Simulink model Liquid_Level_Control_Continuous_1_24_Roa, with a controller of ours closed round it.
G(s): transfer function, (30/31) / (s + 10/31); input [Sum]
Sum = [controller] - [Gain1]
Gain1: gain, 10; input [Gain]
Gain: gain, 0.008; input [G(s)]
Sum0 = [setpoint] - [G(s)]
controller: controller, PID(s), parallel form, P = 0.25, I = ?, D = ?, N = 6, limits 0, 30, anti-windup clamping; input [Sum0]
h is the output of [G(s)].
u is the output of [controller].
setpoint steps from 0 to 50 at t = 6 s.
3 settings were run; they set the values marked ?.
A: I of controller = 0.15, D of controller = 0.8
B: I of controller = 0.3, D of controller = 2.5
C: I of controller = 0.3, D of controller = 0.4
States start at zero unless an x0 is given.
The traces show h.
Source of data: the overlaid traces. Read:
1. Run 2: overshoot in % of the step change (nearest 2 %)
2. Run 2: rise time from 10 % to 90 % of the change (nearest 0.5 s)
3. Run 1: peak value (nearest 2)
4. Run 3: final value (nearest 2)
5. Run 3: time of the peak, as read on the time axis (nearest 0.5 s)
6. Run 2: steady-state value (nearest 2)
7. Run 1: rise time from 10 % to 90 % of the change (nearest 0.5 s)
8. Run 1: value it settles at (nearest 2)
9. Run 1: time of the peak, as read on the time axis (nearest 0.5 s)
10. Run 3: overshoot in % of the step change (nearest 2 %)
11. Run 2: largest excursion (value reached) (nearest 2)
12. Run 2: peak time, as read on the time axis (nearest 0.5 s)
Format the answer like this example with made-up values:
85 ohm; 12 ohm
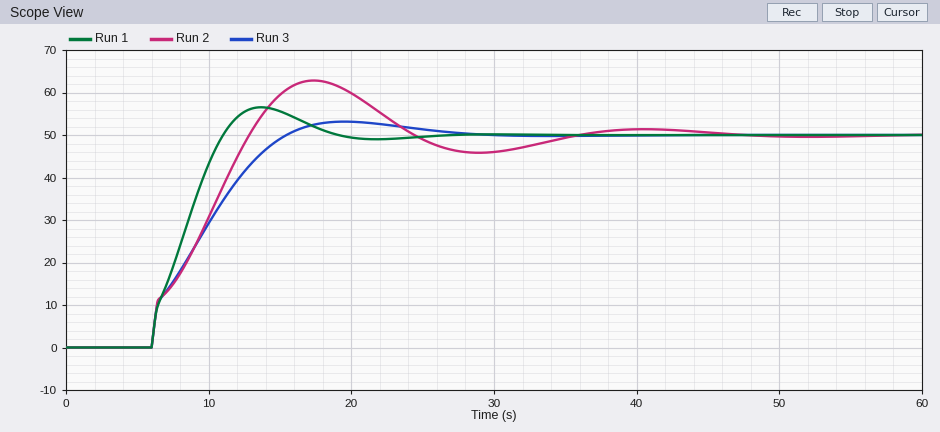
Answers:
26 %; 6.0 s; 56; 50; 19.5 s; 50; 4.0 s; 50; 13.5 s; 6 %; 62; 17.5 s
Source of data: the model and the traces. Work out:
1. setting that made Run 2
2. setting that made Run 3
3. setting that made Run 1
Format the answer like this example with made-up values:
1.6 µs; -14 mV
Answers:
B; A; C
